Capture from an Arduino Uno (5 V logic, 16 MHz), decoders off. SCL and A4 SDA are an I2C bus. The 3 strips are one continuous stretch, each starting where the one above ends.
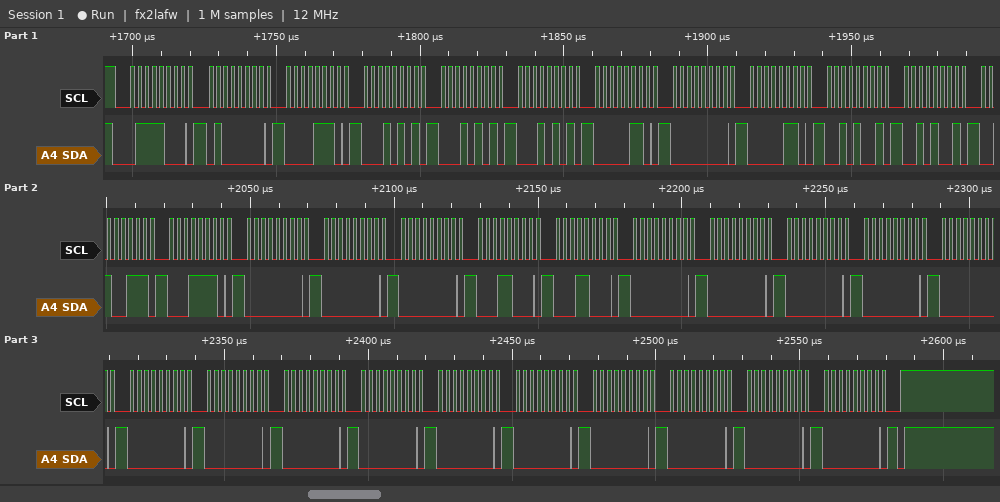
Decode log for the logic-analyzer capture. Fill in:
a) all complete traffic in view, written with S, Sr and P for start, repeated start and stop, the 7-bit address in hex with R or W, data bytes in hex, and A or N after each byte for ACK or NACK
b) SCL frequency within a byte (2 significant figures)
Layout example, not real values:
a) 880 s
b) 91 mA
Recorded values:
a) S 3CW A 40 A 0E A 15 A 15 A 15 A 06 A 00 A 06 A 29 A 29 A 27 A 1E A 00 A 00 A 00 A 18 A 18 A 00 A 00 A 00 A 00 A 00 A 00 A 00 A 00 A 00 A 00 A 00 A 00 A 00 A 00 A 00 A P
b) 400 kHz
